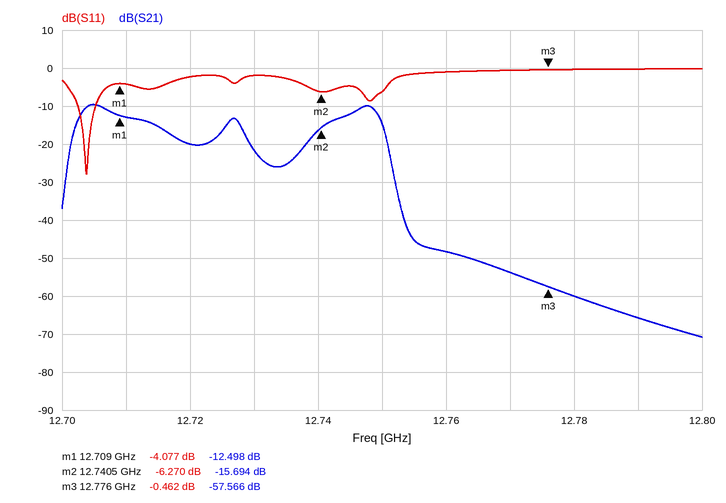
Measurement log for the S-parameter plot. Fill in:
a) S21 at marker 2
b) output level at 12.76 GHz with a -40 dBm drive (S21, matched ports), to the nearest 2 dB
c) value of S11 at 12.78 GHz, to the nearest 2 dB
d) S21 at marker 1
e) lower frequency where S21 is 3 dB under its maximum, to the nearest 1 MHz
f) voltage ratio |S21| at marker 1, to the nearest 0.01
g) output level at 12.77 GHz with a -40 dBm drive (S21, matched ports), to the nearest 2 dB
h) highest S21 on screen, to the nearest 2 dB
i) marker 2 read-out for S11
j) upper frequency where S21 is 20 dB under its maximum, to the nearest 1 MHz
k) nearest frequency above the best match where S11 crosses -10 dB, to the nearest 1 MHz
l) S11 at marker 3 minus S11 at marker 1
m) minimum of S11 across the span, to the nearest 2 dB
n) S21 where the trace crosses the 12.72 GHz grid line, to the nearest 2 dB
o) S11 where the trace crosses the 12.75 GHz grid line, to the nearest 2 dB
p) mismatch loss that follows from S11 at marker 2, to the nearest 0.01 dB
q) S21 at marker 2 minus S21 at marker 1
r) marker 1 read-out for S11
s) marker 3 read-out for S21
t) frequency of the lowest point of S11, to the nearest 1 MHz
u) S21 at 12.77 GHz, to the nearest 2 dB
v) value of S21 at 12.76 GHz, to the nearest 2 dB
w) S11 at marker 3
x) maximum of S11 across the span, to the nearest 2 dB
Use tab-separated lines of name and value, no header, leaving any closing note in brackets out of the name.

S21 at marker 2	-15.694 dB
output level at 12.76 GHz with a -40 dBm drive (S21, matched ports), to the nearest 2 dB	-88 dBm
value of S11 at 12.78 GHz, to the nearest 2 dB	0 dB
S21 at marker 1	-12.498 dB
lower frequency where S21 is 3 dB under its maximum, to the nearest 1 MHz	12.703 GHz
voltage ratio |S21| at marker 1, to the nearest 0.01	0.24
output level at 12.77 GHz with a -40 dBm drive (S21, matched ports), to the nearest 2 dB	-94 dBm
highest S21 on screen, to the nearest 2 dB	-10 dB
marker 2 read-out for S11	-6.270 dB
upper frequency where S21 is 20 dB under its maximum, to the nearest 1 MHz	12.752 GHz
nearest frequency above the best match where S11 crosses -10 dB, to the nearest 1 MHz	12.705 GHz
S11 at marker 3 minus S11 at marker 1	3.615 dB
minimum of S11 across the span, to the nearest 2 dB	-28 dB
S21 where the trace crosses the 12.72 GHz grid line, to the nearest 2 dB	-20 dB
S11 where the trace crosses the 12.75 GHz grid line, to the nearest 2 dB	-6 dB
mismatch loss that follows from S11 at marker 2, to the nearest 0.01 dB	1.17 dB
S21 at marker 2 minus S21 at marker 1	-3.196 dB
marker 1 read-out for S11	-4.077 dB
marker 3 read-out for S21	-57.566 dB
frequency of the lowest point of S11, to the nearest 1 MHz	12.704 GHz
S21 at 12.77 GHz, to the nearest 2 dB	-54 dB
value of S21 at 12.76 GHz, to the nearest 2 dB	-48 dB
S11 at marker 3	-0.462 dB
maximum of S11 across the span, to the nearest 2 dB	0 dB
